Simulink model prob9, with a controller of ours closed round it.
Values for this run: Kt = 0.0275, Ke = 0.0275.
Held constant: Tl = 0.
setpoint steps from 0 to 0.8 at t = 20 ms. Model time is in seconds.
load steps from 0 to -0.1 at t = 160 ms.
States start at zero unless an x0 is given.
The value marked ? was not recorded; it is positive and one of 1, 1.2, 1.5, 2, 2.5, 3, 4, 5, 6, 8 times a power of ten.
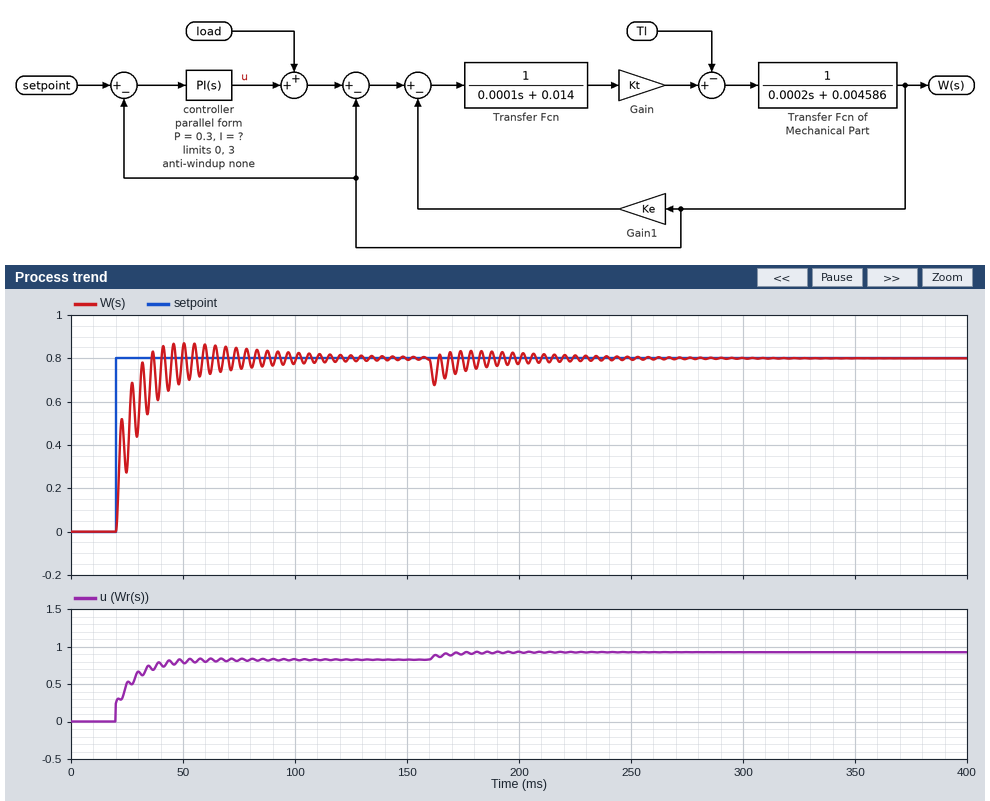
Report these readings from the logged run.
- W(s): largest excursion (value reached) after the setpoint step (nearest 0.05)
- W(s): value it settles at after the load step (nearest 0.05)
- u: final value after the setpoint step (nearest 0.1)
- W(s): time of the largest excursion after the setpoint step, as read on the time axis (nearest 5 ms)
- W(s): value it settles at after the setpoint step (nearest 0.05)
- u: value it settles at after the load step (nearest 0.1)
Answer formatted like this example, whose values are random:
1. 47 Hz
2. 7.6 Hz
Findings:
1. 0.85
2. 0.80
3. 0.8
4. 50 ms
5. 0.80
6. 0.9
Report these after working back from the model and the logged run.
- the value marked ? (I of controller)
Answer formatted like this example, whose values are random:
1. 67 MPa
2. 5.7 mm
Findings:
1. 150
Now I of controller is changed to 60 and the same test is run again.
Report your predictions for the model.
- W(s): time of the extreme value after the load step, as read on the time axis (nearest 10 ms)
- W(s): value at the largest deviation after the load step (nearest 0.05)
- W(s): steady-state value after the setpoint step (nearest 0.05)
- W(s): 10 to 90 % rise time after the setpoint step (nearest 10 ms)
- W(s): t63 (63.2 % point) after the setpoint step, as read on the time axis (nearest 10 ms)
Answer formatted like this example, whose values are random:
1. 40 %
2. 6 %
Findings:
1. 160 ms
2. 0.65
3. 0.80
4. 40 ms
5. 30 ms
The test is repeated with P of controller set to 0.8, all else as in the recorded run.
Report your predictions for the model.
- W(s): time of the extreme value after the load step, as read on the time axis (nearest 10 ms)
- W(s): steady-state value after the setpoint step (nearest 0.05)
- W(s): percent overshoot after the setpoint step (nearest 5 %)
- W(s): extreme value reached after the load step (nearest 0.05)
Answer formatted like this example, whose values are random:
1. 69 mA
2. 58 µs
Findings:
1. 160 ms
2. 0.80
3. 10 %
4. 0.70
